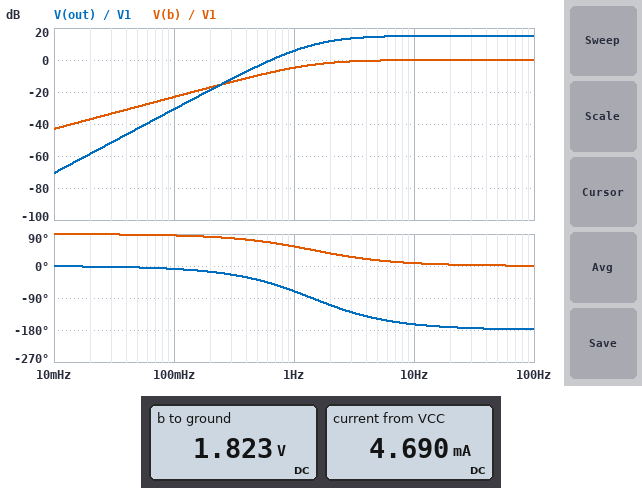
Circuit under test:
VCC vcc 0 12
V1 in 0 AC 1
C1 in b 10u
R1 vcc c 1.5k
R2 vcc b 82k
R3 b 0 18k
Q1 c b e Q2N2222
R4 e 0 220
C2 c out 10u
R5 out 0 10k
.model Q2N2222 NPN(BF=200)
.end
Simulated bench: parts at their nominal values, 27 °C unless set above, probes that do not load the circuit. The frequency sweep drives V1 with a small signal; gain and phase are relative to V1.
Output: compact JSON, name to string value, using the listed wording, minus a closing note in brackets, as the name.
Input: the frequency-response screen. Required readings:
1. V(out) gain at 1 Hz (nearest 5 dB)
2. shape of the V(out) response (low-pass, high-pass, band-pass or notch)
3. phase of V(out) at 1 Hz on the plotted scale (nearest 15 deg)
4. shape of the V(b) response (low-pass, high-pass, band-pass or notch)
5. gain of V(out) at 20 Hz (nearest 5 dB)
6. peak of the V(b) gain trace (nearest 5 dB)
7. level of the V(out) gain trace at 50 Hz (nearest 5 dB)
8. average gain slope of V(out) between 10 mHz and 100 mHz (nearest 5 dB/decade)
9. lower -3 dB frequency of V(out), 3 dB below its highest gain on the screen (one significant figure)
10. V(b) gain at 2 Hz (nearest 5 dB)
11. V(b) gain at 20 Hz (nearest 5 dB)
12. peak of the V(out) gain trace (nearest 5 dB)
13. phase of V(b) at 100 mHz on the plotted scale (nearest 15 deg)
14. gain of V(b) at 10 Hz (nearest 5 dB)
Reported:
{"V(out) gain at 1 Hz": "5 dB", "shape of the V(out) response": "high-pass", "phase of V(out) at 1 Hz on the plotted scale": "-75 deg", "shape of the V(b) response": "high-pass", "gain of V(out) at 20 Hz": "15 dB", "peak of the V(b) gain trace": "0 dB", "level of the V(out) gain trace at 50 Hz": "15 dB", "average gain slope of V(out) between 10 mHz and 100 mHz": "40 dB/decade", "lower -3 dB frequency of V(out), 3 dB below its highest gain on the screen": "2 Hz", "V(b) gain at 2 Hz": "0 dB", "V(b) gain at 20 Hz": "0 dB", "peak of the V(out) gain trace": "15 dB", "phase of V(b) at 100 mHz on the plotted scale": "90 deg", "gain of V(b) at 10 Hz": "0 dB"}
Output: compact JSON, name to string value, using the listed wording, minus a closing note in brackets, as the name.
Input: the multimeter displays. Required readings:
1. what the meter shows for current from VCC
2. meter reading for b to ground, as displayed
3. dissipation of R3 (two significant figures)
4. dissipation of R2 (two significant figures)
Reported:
{"what the meter shows for current from VCC": "4.690 mA", "meter reading for b to ground, as displayed": "1.823 V", "dissipation of R3": "180 µW", "dissipation of R2": "1.3 mW"}
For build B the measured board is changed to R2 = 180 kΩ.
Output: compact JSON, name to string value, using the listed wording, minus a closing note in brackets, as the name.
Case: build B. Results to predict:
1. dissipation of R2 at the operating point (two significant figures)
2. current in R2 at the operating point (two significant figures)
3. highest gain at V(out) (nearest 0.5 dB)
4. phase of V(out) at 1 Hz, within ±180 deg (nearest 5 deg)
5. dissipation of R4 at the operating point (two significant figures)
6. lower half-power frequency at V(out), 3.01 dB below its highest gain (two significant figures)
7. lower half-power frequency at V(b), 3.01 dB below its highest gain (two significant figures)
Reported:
{"dissipation of R2 at the operating point": "670 µW", "current in R2 at the operating point": "61 µA", "highest gain at V(out)": "14.5 dB", "phase of V(out) at 1 Hz, within ±180 deg": "-75 deg", "dissipation of R4 at the operating point": "240 µW", "lower half-power frequency at V(out), 3.01 dB below its highest gain": "2.1 Hz", "lower half-power frequency at V(b), 3.01 dB below its highest gain": "1.3 Hz"}
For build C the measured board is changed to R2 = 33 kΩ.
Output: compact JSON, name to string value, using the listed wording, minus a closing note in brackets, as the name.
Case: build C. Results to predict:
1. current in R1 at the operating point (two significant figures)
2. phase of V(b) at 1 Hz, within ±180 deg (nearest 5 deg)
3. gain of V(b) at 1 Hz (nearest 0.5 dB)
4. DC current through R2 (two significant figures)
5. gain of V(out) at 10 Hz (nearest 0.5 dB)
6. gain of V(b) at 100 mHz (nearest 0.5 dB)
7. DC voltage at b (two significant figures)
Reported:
{"current in R1 at the operating point": "6.9 mA", "phase of V(b) at 1 Hz, within ±180 deg": "90 deg", "gain of V(b) at 1 Hz": "-37.0 dB", "DC current through R2": "290 µA", "gain of V(out) at 10 Hz": "-39.5 dB", "gain of V(b) at 100 mHz": "-57.0 dB", "DC voltage at b": "2.4 V"}
